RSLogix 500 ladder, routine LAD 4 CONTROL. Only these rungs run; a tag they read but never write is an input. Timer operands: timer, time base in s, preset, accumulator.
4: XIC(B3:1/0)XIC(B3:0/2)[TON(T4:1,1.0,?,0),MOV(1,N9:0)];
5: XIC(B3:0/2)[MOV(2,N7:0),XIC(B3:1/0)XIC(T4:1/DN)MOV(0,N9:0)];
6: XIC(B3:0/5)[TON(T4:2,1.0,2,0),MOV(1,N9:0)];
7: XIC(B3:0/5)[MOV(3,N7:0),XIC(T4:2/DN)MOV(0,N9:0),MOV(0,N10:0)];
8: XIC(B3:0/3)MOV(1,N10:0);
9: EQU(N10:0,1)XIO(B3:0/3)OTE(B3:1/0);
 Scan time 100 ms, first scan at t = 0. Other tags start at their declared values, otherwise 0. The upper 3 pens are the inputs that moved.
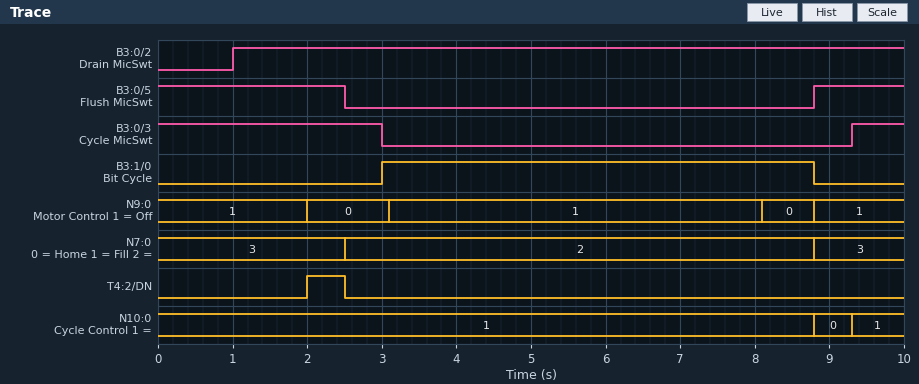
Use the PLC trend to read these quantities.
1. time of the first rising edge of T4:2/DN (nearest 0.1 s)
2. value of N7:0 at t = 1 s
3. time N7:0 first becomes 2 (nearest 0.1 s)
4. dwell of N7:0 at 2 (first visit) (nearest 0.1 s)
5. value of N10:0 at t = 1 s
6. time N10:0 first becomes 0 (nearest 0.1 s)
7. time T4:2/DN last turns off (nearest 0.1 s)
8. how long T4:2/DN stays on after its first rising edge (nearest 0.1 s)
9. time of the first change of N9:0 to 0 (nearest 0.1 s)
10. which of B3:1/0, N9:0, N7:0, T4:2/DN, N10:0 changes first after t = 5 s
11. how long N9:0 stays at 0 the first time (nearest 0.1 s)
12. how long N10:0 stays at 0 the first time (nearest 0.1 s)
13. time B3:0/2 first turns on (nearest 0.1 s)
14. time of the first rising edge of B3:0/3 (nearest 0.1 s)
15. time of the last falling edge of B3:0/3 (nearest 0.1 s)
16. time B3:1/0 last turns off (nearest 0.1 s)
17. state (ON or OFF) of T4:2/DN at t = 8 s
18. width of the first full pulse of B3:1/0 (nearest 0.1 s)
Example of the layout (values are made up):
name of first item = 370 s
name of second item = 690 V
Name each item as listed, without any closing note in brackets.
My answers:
time of the first rising edge of T4:2/DN = 2.0 s
value of N7:0 at t = 1 s = 3
time N7:0 first becomes 2 = 2.5 s
dwell of N7:0 at 2 (first visit) = 6.3 s
value of N10:0 at t = 1 s = 1
time N10:0 first becomes 0 = 8.8 s
time T4:2/DN last turns off = 2.5 s
how long T4:2/DN stays on after its first rising edge = 0.5 s
time of the first change of N9:0 to 0 = 2.0 s
which of B3:1/0, N9:0, N7:0, T4:2/DN, N10:0 changes first after t = 5 s = N9:0
how long N9:0 stays at 0 the first time = 1.1 s
how long N10:0 stays at 0 the first time = 0.5 s
time B3:0/2 first turns on = 1.0 s
time of the first rising edge of B3:0/3 = 9.3 s
time of the last falling edge of B3:0/3 = 3.0 s
time B3:1/0 last turns off = 8.8 s
state (ON or OFF) of T4:2/DN at t = 8 s = OFF
width of the first full pulse of B3:1/0 = 5.8 s
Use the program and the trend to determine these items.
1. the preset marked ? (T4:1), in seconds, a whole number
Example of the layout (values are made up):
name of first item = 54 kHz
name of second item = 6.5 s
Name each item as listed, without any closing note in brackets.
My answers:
the preset marked ? (T4:1), in seconds, a whole number = 5 s
